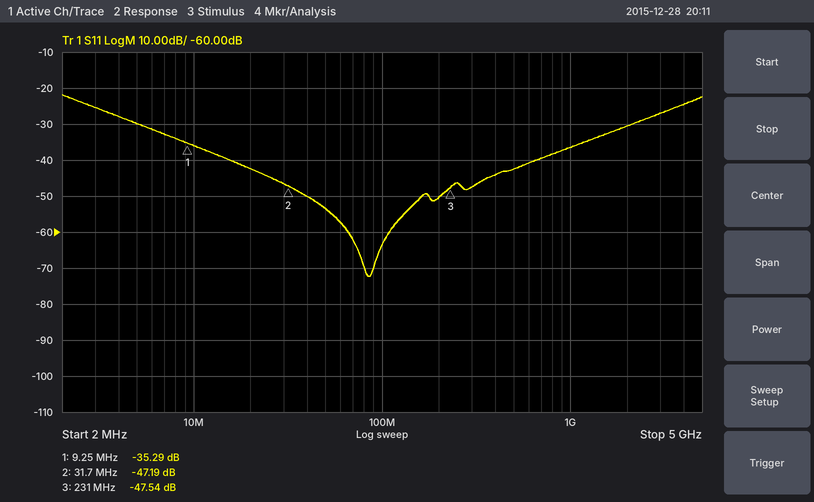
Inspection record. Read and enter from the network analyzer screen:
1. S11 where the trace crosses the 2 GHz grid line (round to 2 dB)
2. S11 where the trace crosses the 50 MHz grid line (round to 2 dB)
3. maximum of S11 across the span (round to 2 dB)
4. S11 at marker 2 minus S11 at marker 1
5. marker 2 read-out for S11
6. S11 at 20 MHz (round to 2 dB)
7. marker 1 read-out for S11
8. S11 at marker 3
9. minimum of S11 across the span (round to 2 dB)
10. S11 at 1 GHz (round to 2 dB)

-30 dB
-54 dB
-22 dB
-11.90 dB
-47.19 dB
-42 dB
-35.29 dB
-47.54 dB
-72 dB
-36 dB
